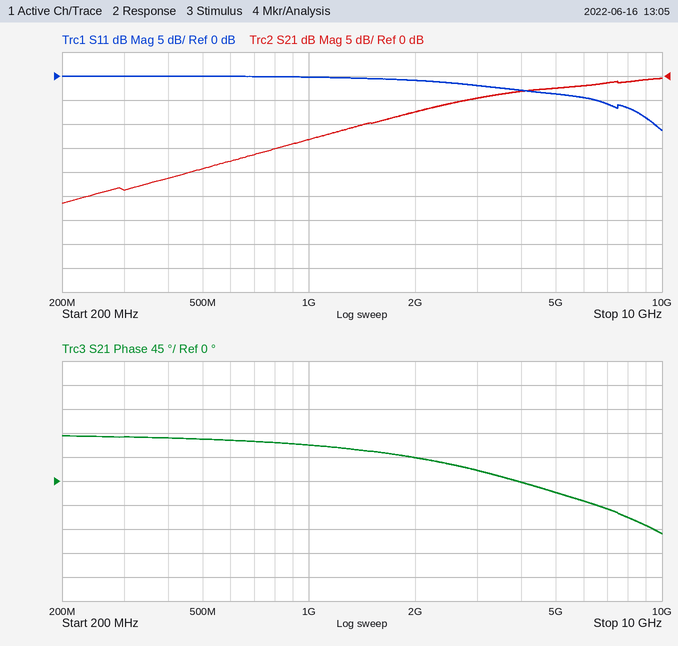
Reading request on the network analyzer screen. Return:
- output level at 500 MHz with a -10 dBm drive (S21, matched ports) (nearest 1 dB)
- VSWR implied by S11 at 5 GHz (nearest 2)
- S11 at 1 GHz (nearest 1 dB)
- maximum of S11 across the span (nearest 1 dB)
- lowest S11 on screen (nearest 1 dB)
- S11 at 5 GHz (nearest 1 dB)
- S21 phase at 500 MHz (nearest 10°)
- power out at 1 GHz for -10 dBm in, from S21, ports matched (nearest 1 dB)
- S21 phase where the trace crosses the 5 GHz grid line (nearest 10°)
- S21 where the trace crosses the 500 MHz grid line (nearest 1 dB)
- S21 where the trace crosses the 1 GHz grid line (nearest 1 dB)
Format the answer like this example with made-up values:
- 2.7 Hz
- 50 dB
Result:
- -29 dBm
- 4
- 0 dB
- 0 dB
- -11 dB
- -4 dB
- 80°
- -23 dBm
- -20°
- -19 dB
- -13 dB
